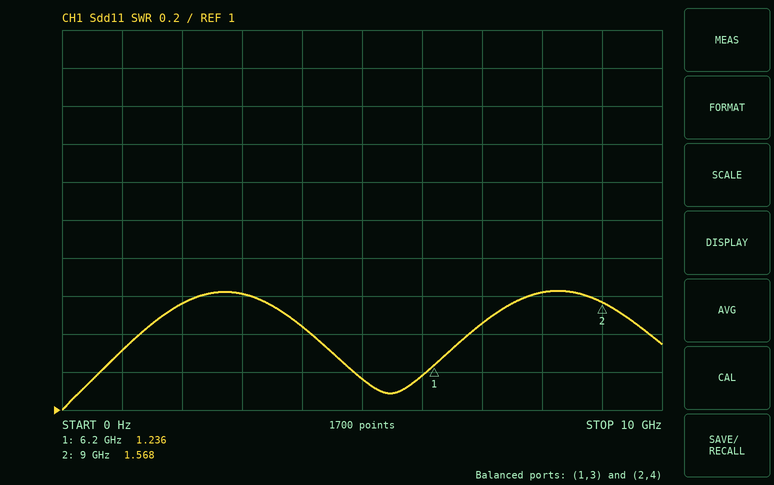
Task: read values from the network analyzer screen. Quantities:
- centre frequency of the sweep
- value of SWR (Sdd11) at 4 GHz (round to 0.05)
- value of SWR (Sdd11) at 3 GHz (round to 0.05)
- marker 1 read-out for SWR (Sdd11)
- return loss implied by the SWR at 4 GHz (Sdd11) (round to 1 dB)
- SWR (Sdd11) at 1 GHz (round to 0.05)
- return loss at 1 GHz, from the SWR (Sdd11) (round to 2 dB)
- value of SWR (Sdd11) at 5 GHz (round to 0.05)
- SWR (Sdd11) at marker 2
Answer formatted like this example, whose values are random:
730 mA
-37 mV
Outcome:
5 GHz
1.45
1.60
1.236
15 dB
1.30
18 dB
1.15
1.568
